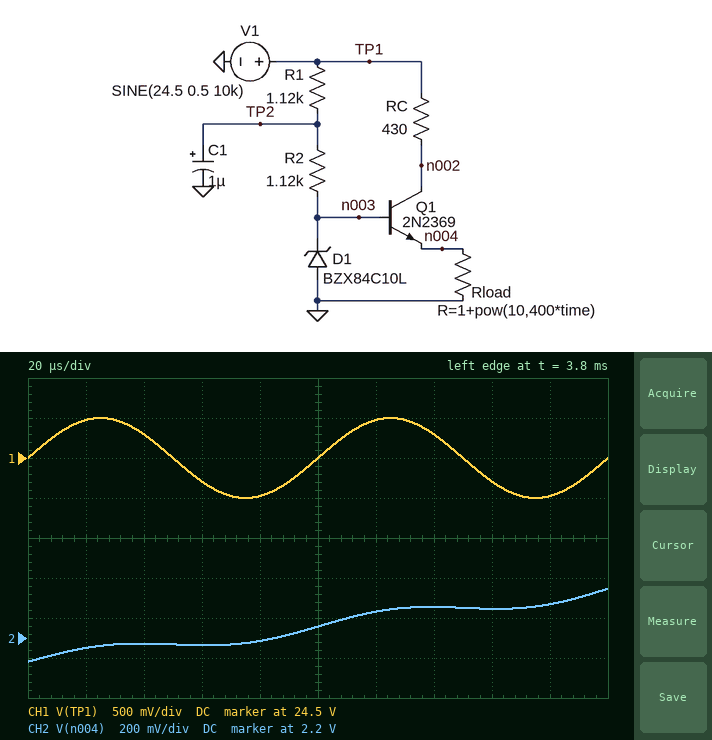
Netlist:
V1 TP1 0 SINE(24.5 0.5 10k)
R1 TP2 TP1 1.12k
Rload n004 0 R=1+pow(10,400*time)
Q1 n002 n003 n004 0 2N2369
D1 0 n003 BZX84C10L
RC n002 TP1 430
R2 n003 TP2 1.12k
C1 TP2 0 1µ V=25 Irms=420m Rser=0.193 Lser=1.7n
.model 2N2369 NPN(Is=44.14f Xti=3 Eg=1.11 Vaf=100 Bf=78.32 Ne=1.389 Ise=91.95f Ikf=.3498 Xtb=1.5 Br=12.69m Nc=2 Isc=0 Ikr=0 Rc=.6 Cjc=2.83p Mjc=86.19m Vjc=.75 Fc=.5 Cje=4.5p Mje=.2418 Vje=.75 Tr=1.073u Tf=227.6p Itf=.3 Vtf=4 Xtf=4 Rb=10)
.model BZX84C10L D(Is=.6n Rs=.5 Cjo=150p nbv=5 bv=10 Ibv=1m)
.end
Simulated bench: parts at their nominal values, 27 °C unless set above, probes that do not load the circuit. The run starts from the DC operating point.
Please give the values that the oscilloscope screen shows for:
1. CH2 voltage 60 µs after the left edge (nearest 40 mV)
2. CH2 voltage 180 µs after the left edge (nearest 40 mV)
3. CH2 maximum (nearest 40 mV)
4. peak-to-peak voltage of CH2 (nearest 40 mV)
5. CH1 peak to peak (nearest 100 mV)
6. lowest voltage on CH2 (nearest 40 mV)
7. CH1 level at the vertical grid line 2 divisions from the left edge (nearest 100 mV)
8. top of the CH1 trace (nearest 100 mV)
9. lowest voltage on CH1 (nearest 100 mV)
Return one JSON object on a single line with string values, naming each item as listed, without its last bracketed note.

{"CH2 voltage 60 µs after the left edge": "2.16 V", "CH2 voltage 180 µs after the left edge": "2.36 V", "CH2 maximum": "2.44 V", "peak-to-peak voltage of CH2": "360 mV", "CH1 peak to peak": "1.0 V", "lowest voltage on CH2": "2.08 V", "CH1 level at the vertical grid line 2 divisions from the left edge": "24.8 V", "top of the CH1 trace": "25.0 V", "lowest voltage on CH1": "24.0 V"}
